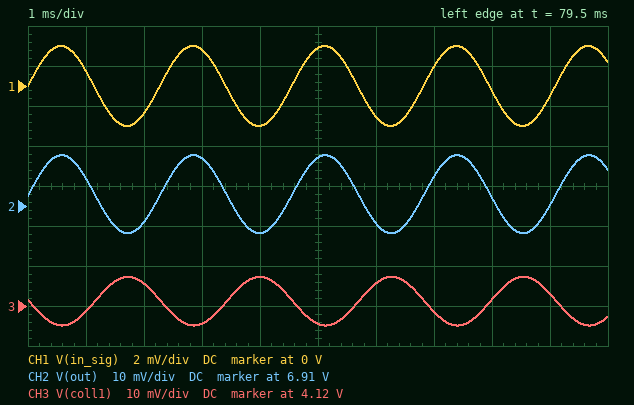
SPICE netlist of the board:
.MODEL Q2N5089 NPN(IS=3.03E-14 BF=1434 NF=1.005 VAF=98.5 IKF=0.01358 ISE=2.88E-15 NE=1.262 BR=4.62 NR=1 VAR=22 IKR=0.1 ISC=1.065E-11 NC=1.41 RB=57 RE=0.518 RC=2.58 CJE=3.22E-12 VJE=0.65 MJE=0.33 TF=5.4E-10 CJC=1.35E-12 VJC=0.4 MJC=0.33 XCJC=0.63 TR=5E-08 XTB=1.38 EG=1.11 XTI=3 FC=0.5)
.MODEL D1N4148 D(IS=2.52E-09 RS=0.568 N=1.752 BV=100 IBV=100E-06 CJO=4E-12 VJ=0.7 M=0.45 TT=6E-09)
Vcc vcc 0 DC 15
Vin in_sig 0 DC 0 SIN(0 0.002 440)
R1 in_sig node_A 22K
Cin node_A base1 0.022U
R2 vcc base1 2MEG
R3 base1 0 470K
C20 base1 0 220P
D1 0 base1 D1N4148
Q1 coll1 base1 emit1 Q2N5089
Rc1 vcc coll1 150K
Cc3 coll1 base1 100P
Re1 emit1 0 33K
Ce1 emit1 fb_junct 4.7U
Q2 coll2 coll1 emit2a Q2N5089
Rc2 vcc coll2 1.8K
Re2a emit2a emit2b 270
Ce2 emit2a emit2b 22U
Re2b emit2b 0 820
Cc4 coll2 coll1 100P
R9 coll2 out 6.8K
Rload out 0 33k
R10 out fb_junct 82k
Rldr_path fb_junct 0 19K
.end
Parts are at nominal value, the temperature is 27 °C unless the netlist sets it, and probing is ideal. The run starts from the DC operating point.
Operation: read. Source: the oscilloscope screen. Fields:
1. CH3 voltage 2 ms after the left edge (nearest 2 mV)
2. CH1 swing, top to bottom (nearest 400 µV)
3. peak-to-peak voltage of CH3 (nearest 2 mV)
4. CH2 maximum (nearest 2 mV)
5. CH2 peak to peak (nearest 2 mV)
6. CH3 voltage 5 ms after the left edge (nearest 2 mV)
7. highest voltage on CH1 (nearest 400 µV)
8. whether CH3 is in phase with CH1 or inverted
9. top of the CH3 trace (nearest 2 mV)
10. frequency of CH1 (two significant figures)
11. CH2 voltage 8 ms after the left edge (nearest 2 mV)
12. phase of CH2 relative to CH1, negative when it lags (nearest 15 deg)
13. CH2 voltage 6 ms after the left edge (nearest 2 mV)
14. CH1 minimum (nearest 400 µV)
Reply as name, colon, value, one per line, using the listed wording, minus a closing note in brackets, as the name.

CH3 voltage 2 ms after the left edge: 4.126 V
CH1 swing, top to bottom: 4.0 mV
peak-to-peak voltage of CH3: 12 mV
CH2 maximum: 6.922 V
CH2 peak to peak: 20 mV
CH3 voltage 5 ms after the left edge: 4.116 V
highest voltage on CH1: 2.0 mV
whether CH3 is in phase with CH1 or inverted: inverted
top of the CH3 trace: 4.128 V
frequency of CH1: 440 Hz
CH2 voltage 8 ms after the left edge: 6.912 V
phase of CH2 relative to CH1, negative when it lags: 0 deg
CH2 voltage 6 ms after the left edge: 6.906 V
CH1 minimum: -2.0 mV
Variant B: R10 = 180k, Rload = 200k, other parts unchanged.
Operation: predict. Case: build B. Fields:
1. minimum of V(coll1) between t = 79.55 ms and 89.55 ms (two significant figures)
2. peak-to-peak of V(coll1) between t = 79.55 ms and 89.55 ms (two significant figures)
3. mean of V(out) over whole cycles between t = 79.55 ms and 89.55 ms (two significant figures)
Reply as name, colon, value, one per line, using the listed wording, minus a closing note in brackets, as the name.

minimum of V(coll1) between t = 79.55 ms and 89.55 ms: 4.1 V
peak-to-peak of V(coll1) between t = 79.55 ms and 89.55 ms: 16 mV
mean of V(out) over whole cycles between t = 79.55 ms and 89.55 ms: 8.6 V
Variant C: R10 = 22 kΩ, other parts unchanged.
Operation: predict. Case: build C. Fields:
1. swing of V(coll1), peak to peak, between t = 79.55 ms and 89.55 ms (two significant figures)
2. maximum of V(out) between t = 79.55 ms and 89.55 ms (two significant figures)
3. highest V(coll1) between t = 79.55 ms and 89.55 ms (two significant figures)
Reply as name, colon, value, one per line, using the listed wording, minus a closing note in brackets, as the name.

swing of V(coll1), peak to peak, between t = 79.55 ms and 89.55 ms: 6.3 mV
maximum of V(out) between t = 79.55 ms and 89.55 ms: 6.3 V
highest V(coll1) between t = 79.55 ms and 89.55 ms: 4.1 V
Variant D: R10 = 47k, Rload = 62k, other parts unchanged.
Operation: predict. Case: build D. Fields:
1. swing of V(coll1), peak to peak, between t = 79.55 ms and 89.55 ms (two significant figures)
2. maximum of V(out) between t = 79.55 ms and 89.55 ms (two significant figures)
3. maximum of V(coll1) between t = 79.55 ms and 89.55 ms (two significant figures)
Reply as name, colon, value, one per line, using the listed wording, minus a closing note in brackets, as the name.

swing of V(coll1), peak to peak, between t = 79.55 ms and 89.55 ms: 8.5 mV
maximum of V(out) between t = 79.55 ms and 89.55 ms: 7.3 V
maximum of V(coll1) between t = 79.55 ms and 89.55 ms: 4.1 V
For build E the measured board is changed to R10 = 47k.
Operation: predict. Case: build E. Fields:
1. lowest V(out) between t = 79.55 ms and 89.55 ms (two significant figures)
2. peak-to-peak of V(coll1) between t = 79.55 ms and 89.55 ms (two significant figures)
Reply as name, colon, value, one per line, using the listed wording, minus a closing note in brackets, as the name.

lowest V(out) between t = 79.55 ms and 89.55 ms: 6.7 V
peak-to-peak of V(coll1) between t = 79.55 ms and 89.55 ms: 9.1 mV
